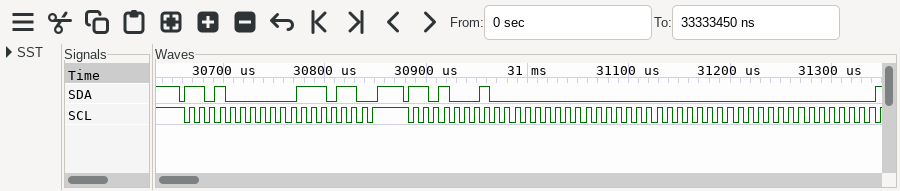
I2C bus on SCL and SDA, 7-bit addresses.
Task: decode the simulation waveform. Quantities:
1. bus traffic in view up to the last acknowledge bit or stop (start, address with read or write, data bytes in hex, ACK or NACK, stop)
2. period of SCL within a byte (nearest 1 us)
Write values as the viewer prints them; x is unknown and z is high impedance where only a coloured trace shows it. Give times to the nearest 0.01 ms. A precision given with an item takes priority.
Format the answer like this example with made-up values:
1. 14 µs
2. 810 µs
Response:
1. start, address 68 write ACK, 3B ACK, stop, start, address 68 read ACK, 00 ACK, 00 ACK, 00 ACK, 00 ACK
2. 10 us
